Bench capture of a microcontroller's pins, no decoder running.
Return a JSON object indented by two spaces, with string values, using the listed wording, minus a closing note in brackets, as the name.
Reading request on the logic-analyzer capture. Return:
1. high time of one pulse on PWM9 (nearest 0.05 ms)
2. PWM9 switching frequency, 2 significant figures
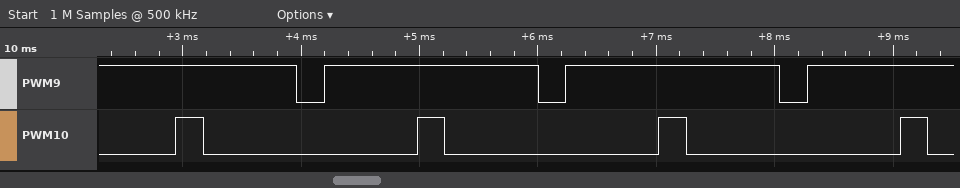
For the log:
{
  "high time of one pulse on PWM9": "1.80 ms",
  "PWM9 switching frequency, 2 significant figures": "490 Hz"
}
